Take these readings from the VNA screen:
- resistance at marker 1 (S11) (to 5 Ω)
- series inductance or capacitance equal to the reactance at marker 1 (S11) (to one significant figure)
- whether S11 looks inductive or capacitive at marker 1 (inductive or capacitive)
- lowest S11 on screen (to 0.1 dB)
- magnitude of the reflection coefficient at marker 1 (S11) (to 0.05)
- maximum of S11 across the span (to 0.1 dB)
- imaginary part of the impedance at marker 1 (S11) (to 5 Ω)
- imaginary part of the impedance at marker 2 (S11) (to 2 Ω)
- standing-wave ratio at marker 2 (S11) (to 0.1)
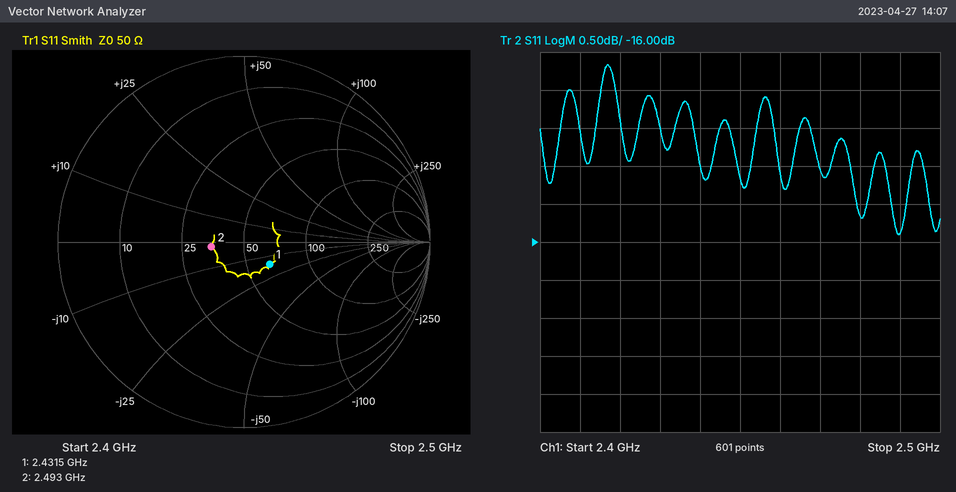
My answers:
65 Ω
4 pF
capacitive
-15.9 dB
0.20
-13.7 dB
-15 Ω
-2 Ω
1.4
